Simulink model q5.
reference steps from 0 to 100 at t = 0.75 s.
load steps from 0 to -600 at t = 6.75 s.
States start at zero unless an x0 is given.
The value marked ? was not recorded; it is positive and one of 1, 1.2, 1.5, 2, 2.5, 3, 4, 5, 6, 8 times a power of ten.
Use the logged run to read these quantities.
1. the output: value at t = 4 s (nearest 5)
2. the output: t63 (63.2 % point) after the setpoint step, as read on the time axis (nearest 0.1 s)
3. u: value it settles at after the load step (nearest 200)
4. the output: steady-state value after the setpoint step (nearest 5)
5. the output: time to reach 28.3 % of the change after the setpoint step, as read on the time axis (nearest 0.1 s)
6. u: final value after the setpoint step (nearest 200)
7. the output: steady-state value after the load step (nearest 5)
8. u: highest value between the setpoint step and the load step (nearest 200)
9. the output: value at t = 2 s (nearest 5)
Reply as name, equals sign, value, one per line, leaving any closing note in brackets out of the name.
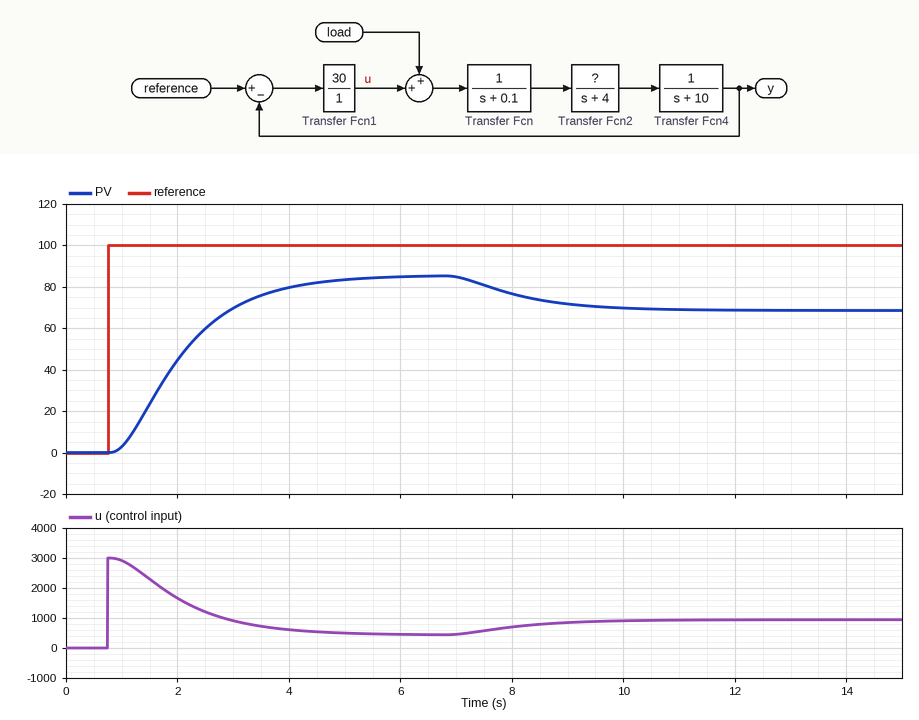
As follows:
the output: value at t = 4 s = 80
the output: t63 (63.2 % point) after the setpoint step, as read on the time axis = 2.3 s
u: value it settles at after the load step = 1000
the output: steady-state value after the setpoint step = 85
the output: time to reach 28.3 % of the change after the setpoint step, as read on the time axis = 1.5 s
u: final value after the setpoint step = 400
the output: steady-state value after the load step = 70
u: highest value between the setpoint step and the load step = 3000
the output: value at t = 2 s = 45
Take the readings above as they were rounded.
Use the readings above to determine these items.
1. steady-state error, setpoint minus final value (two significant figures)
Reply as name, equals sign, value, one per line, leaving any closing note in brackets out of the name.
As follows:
steady-state error, setpoint minus final value = 15
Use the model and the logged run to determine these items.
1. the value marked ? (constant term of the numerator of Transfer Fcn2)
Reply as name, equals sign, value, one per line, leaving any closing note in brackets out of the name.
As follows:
the value marked ? = 0.8
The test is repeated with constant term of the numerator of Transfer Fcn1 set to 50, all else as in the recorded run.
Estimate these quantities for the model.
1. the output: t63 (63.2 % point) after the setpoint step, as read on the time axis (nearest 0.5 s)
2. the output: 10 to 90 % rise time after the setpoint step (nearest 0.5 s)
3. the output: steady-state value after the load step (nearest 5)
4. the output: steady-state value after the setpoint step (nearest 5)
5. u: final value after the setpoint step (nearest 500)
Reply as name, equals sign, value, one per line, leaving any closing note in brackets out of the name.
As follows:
the output: t63 (63.2 % point) after the setpoint step, as read on the time axis = 2.0 s
the output: 10 to 90 % rise time after the setpoint step = 1.5 s
the output: steady-state value after the load step = 80
the output: steady-state value after the setpoint step = 90
u: final value after the setpoint step = 500
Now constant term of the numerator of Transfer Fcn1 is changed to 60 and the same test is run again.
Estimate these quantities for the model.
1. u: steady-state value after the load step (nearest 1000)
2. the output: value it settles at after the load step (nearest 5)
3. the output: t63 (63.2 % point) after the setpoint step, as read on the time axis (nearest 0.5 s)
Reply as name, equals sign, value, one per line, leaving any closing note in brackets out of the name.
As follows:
u: steady-state value after the load step = 1000
the output: value it settles at after the load step = 85
the output: t63 (63.2 % point) after the setpoint step, as read on the time axis = 1.5 s
